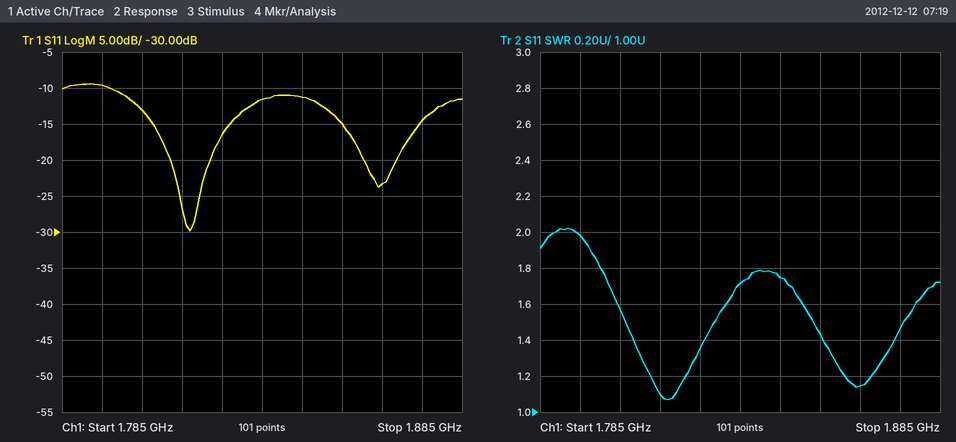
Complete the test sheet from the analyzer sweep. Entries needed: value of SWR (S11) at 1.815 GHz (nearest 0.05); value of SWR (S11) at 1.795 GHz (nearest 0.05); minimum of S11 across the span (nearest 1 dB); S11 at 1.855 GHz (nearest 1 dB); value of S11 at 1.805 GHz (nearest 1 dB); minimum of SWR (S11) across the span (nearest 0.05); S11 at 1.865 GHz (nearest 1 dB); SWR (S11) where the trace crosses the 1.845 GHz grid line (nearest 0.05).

1.10
2.00
-30 dB
-15 dB
-13 dB
1.05
-23 dB
1.75
